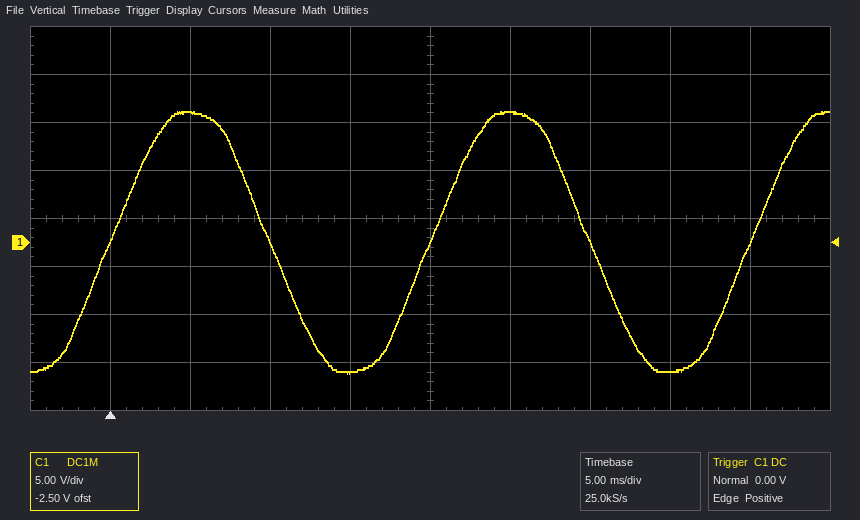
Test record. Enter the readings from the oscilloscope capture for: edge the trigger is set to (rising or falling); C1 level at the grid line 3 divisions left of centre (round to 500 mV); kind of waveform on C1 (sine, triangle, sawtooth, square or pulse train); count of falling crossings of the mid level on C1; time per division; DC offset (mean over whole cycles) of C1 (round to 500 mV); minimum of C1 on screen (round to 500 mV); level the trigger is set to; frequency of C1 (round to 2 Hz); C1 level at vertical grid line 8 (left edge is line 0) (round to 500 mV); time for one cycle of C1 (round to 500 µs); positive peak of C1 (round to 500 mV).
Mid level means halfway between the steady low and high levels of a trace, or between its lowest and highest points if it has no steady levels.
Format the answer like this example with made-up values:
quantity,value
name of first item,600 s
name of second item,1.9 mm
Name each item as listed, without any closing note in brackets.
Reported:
quantity,value
edge the trigger is set to,rising
C1 level at the grid line 3 divisions left of centre,13.5 V
kind of waveform on C1,sine
count of falling crossings of the mid level on C1,2
time per division,5 ms
DC offset (mean over whole cycles) of C1,0.0 V
minimum of C1 on screen,-13.5 V
level the trigger is set to,0.00 V
frequency of C1,50 Hz
C1 level at vertical grid line 8 (left edge is line 0),-13.5 V
time for one cycle of C1,20.0 ms
positive peak of C1,13.5 V
